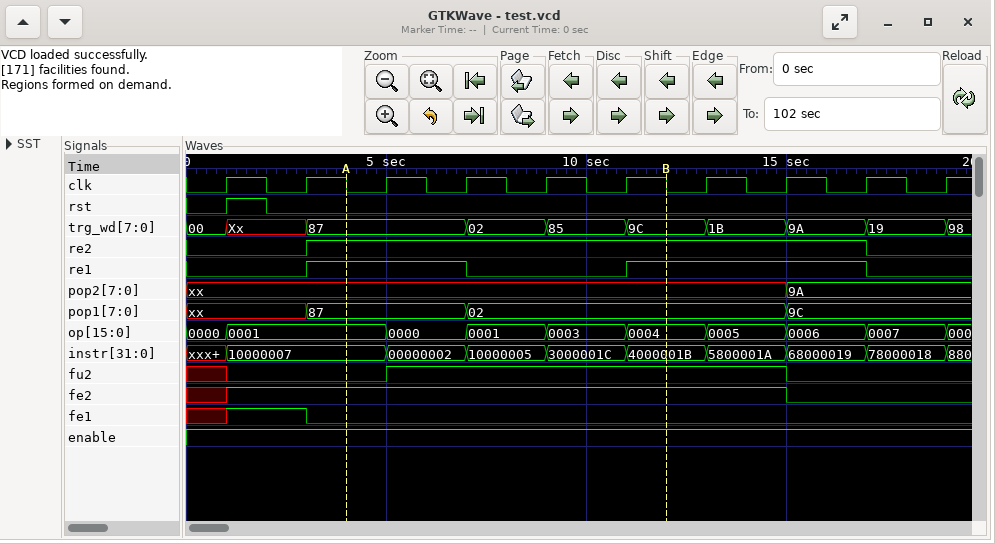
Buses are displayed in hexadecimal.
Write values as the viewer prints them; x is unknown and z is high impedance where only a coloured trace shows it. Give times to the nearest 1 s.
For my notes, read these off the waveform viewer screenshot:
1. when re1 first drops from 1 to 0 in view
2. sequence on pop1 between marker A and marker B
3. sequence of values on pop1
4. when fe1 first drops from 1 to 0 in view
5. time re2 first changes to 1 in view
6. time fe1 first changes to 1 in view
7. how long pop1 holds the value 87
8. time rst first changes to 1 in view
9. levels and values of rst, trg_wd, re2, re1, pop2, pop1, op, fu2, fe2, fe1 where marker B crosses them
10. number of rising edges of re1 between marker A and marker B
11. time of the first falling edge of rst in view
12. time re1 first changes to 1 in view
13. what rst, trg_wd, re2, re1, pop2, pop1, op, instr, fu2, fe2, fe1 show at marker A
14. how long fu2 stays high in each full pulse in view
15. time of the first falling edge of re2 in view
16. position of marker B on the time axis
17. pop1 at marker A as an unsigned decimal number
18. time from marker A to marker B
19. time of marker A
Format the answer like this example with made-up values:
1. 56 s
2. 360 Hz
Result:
1. 7 s
2. 87, 02
3. xx, 87, 02, 9C
4. 3 s
5. 3 s
6. 1 s
7. 4 s
8. 1 s
9. rst=0, trg_wd=9C, re2=1, re1=1, pop2=xx, pop1=02, op=0004, fu2=1, fe2=1, fe1=0
10. 1
11. 2 s
12. 3 s
13. rst=0, trg_wd=87, re2=1, re1=1, pop2=xx, pop1=87, op=0001, instr=10000007, fu2=0, fe2=1, fe1=0
14. 10 s
15. 17 s
16. 12 s
17. 135
18. 8 s
19. 4 s
